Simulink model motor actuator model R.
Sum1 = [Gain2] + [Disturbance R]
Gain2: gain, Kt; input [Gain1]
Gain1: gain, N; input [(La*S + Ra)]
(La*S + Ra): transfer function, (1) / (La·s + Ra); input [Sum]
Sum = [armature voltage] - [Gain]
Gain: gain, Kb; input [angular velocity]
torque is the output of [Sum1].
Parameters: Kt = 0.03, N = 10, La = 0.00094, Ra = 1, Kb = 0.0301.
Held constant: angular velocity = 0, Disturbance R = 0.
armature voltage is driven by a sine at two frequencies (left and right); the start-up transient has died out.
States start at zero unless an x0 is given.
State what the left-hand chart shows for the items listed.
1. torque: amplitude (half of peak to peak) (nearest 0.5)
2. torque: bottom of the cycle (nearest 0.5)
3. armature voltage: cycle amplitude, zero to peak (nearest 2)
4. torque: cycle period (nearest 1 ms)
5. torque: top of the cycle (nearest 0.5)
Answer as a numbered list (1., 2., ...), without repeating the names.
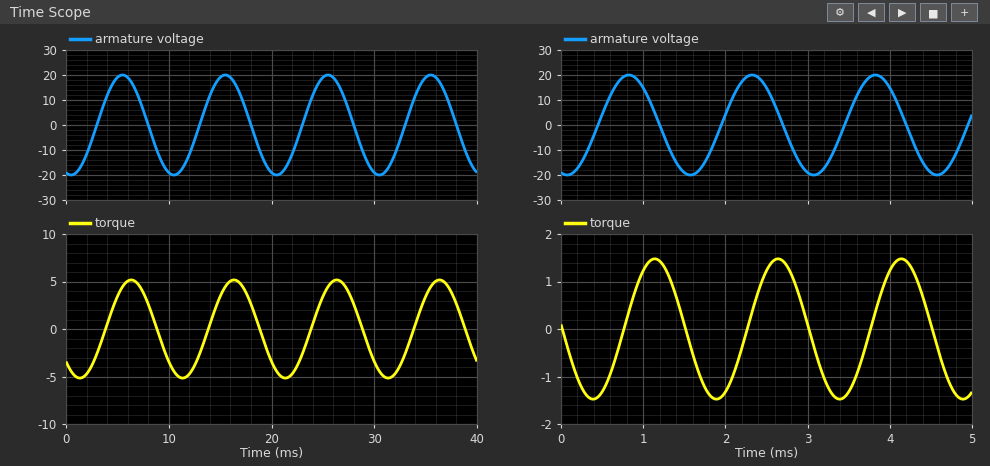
1. 5.0
2. -5.0
3. 20
4. 10 ms
5. 5.0
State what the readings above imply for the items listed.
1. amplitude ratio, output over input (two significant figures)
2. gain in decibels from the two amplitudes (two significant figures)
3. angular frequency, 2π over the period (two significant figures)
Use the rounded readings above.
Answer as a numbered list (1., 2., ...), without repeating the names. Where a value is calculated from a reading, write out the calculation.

1. 5 / 20 = 0.25
2. 20 log10(5 / 20) = -12 dB
3. 2π / 10 = 0.63 rad/ms
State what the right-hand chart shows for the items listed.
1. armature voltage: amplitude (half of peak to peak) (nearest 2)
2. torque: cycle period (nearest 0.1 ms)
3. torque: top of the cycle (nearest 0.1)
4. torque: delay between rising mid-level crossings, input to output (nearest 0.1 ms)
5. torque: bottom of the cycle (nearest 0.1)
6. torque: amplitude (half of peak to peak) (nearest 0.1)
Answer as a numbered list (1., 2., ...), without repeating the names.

1. 20
2. 1.5 ms
3. 1.5
4. 0.3 ms
5. -1.5
6. 1.5
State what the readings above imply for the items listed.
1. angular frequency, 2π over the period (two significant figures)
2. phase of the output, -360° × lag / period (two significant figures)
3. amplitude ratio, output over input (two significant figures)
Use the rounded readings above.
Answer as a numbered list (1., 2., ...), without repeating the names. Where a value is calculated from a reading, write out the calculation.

1. 2π / 1.5 = 4.2 rad/ms
2. -360 × 0.3 / 1.5 = -72°
3. 1.5 / 20 = 0.075
